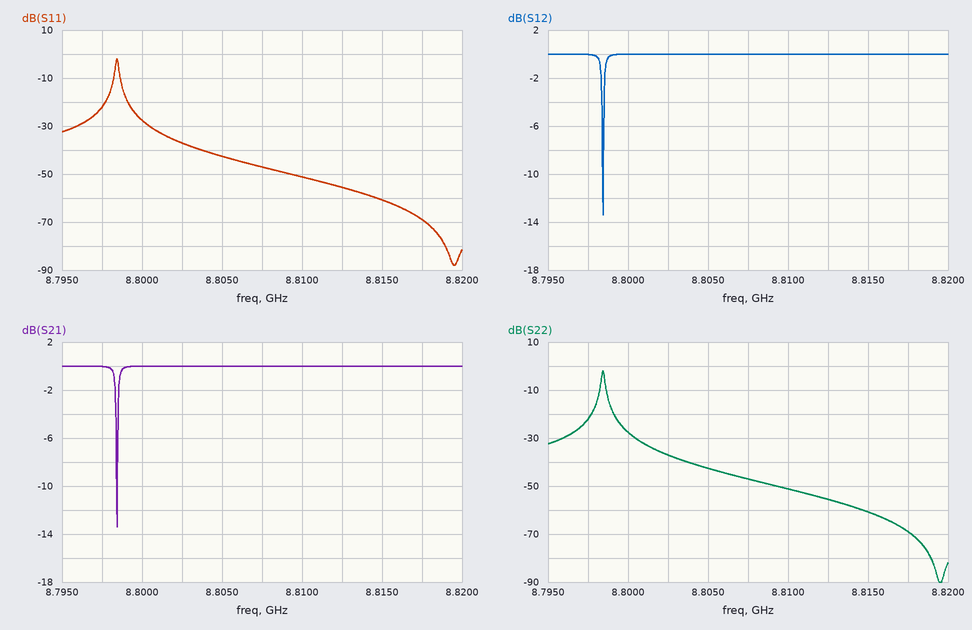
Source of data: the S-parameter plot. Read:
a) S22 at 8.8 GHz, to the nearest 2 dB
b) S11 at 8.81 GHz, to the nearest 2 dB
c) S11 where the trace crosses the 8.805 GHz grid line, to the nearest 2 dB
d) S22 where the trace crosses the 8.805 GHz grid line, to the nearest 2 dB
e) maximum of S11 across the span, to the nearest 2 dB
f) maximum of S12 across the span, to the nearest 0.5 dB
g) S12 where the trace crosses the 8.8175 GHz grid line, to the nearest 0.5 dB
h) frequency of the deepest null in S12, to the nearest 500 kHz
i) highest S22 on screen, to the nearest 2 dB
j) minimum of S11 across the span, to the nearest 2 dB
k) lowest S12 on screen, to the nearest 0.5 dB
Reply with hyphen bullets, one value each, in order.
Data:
- -28 dB
- -52 dB
- -42 dB
- -42 dB
- -2 dB
- 0.0 dB
- 0.0 dB
- 8.7985 GHz
- -2 dB
- -88 dB
- -13.5 dB
